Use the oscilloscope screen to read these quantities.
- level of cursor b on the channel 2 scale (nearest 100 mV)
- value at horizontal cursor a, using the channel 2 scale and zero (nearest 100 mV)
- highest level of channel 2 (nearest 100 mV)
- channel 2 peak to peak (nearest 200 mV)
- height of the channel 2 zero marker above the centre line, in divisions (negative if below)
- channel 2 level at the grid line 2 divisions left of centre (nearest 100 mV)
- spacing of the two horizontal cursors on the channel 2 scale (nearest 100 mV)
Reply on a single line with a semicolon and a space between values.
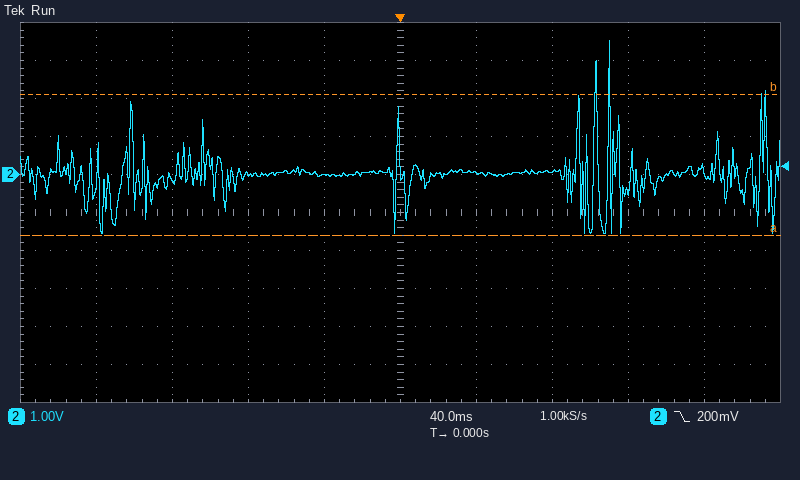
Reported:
2.1 V; -1.6 V; 3.5 V; 5.0 V; +1.0 div; 0.0 V; 3.7 V
